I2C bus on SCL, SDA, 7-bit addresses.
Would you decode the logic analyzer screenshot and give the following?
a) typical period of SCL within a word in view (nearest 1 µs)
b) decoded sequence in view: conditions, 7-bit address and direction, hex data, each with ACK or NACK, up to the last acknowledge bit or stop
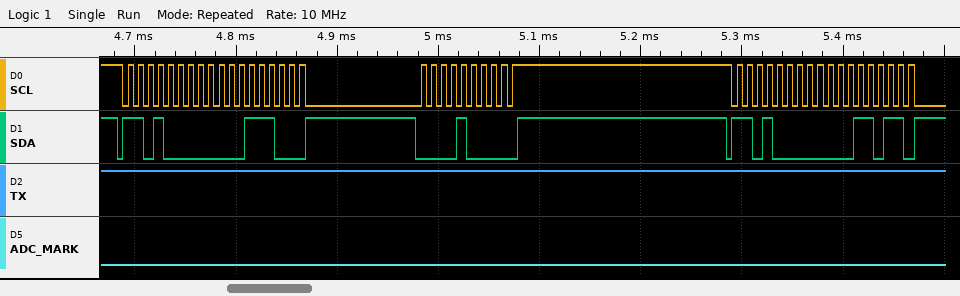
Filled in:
10 µs
start, address 68 write ACK, 1C ACK, 08 ACK, stop, start, address 68 write ACK, 1B ACK
